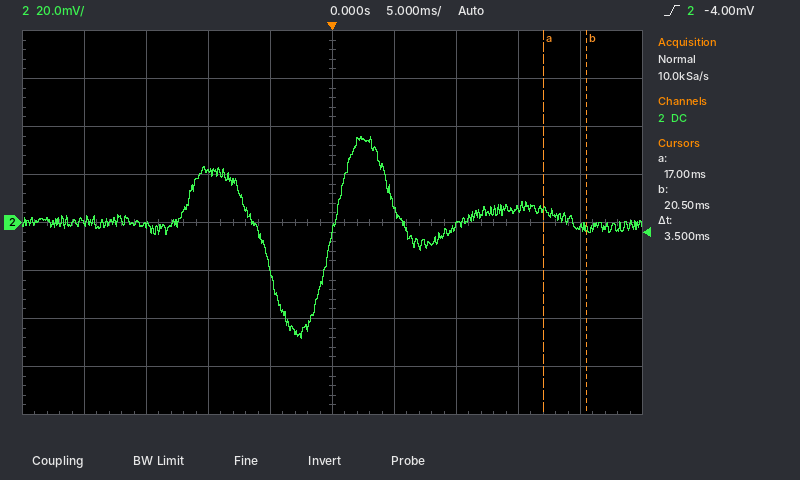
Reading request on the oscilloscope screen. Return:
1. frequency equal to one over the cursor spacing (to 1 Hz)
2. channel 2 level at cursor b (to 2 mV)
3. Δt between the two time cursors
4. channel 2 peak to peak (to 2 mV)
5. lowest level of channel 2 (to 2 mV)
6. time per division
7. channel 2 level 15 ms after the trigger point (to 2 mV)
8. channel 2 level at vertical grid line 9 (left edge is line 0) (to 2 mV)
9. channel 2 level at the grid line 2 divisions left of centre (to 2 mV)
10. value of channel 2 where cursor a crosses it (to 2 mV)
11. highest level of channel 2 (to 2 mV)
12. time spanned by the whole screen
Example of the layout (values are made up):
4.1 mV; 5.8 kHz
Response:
286 Hz; -2 mV; 3.5 ms; 84 mV; -48 mV; 5 ms; 6 mV; -2 mV; 22 mV; 6 mV; 36 mV; 50 ms
